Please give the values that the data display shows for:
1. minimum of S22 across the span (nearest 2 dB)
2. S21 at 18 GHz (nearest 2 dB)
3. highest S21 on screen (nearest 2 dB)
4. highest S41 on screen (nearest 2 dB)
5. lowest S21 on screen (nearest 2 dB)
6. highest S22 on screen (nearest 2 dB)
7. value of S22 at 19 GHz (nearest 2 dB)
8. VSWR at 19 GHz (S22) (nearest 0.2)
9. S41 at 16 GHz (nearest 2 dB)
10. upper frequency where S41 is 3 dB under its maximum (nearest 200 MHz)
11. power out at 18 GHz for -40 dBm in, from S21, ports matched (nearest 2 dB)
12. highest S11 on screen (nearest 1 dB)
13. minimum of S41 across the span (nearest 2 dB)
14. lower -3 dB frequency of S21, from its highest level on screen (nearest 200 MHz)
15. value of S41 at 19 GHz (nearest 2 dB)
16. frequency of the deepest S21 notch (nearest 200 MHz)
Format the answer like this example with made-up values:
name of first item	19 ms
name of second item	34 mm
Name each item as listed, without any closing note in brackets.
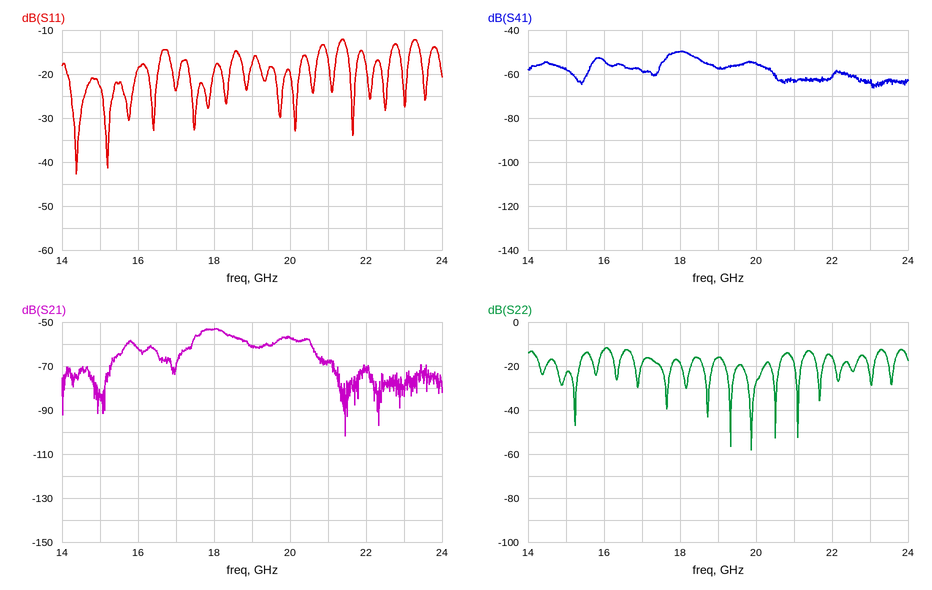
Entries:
minimum of S22 across the span	-58 dB
S21 at 18 GHz	-54 dB
highest S21 on screen	-52 dB
highest S41 on screen	-50 dB
lowest S21 on screen	-102 dB
highest S22 on screen	-12 dB
value of S22 at 19 GHz	-16 dB
VSWR at 19 GHz (S22)	1.4
S41 at 16 GHz	-54 dB
upper frequency where S41 is 3 dB under its maximum	18.4 GHz
power out at 18 GHz for -40 dBm in, from S21, ports matched	-94 dBm
highest S11 on screen	-12 dB
minimum of S41 across the span	-66 dB
lower -3 dB frequency of S21, from its highest level on screen	17.6 GHz
value of S41 at 19 GHz	-58 dB
frequency of the deepest S21 notch	21.4 GHz
